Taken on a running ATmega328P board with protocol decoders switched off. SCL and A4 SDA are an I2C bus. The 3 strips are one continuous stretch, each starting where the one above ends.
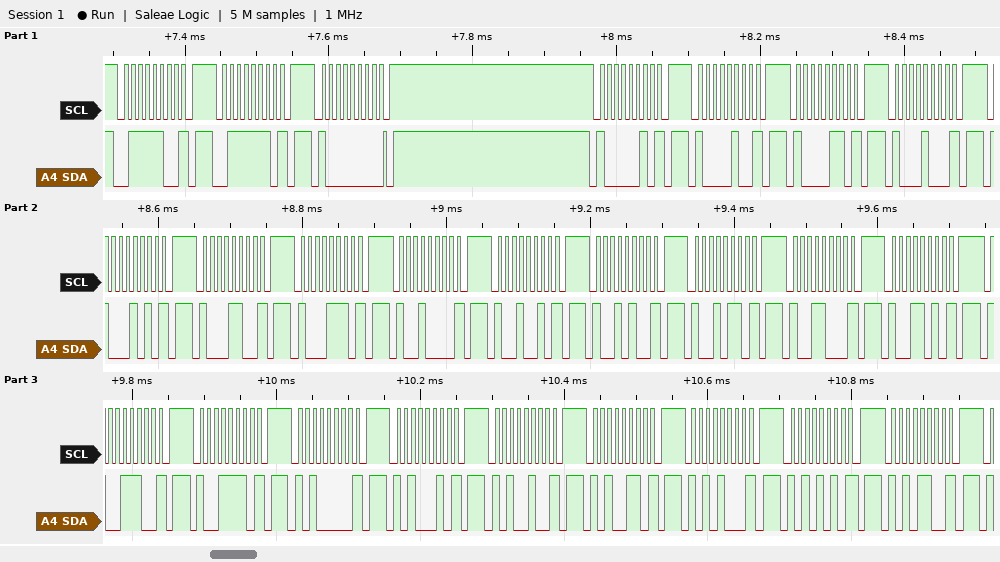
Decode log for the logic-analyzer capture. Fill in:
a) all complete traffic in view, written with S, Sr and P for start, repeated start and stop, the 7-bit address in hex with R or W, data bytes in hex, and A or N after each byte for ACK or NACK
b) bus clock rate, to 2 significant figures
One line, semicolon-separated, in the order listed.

S 3EW N P S 3FW N P S 40W A P S 41W N P S 42W N P S 43W N P S 44W N P S 45W N P S 46W N P S 47W N P S 48W N P S 49W N P S 4AW N P S 4BW N P S 4CW N P S 4DW N P S 4EW N P S 4FW N P S 50W N P S 51W N P S 52W N P S 53W N P S 54W N P S 55W N P S 56W N P; 100 kHz
